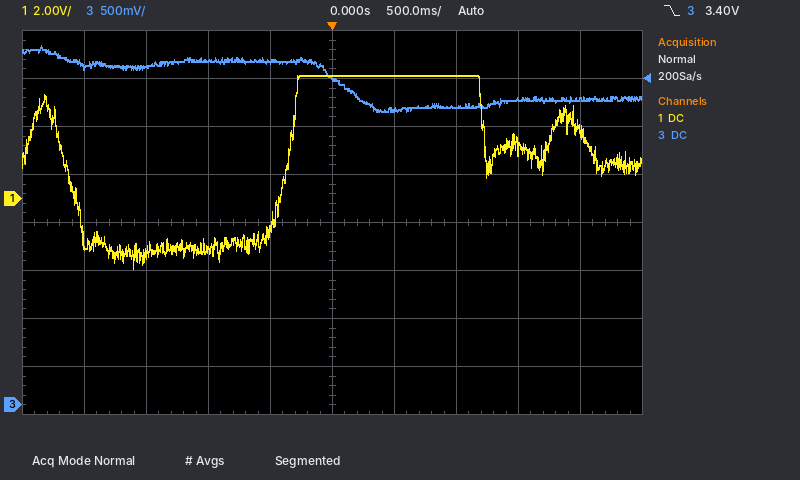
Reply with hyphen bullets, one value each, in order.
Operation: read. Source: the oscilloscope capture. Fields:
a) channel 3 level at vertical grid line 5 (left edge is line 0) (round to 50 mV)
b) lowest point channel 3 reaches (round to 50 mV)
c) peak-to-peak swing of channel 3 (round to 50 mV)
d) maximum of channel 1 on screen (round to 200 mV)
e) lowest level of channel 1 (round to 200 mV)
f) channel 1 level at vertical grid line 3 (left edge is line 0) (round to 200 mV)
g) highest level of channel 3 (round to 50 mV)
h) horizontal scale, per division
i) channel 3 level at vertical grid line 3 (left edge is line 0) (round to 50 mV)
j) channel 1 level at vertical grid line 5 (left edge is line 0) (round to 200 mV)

- 3.40 V
- 3.05 V
- 700 mV
- 5.2 V
- -3.0 V
- -2.2 V
- 3.75 V
- 500 ms
- 3.60 V
- 5.2 V
